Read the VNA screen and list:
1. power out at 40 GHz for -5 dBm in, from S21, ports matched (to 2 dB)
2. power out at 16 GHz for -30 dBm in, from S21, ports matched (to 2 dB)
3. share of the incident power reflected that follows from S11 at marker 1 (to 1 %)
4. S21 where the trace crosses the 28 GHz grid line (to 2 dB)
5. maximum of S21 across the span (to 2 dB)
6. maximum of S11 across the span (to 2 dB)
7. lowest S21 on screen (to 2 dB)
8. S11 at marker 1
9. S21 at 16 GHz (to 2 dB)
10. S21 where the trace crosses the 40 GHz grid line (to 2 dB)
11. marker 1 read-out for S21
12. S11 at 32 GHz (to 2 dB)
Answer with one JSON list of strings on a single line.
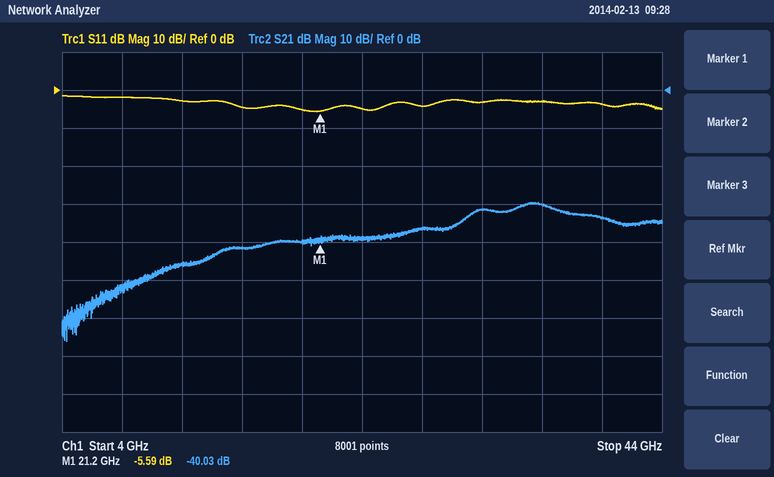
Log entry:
["-38 dBm", "-72 dBm", "28 %", "-36 dB", "-30 dB", "-2 dB", "-66 dB", "-5.59 dB", "-42 dB", "-34 dB", "-40.03 dB", "-4 dB"]
